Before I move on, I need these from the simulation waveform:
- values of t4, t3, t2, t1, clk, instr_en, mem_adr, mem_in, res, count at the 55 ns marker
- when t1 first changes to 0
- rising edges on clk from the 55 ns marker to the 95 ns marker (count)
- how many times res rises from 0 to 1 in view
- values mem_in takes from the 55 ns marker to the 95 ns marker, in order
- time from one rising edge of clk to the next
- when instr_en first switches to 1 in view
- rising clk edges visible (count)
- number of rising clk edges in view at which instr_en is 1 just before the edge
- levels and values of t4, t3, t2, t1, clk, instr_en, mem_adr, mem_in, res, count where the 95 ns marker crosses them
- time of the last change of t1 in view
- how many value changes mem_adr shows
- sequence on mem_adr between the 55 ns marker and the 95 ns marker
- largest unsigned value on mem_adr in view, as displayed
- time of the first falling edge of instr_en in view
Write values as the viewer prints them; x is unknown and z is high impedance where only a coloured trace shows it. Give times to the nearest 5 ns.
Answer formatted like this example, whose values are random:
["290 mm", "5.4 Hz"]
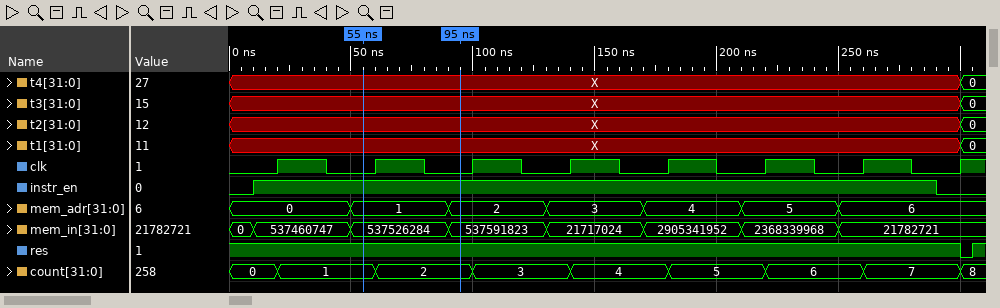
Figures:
["t4=X, t3=X, t2=X, t1=X, clk=0, instr_en=1, mem_adr=1, mem_in=537526284, res=1, count=1", "300 ns", "1", "1", "537526284, 537591823", "40 ns", "10 ns", "8", "7", "t4=X, t3=X, t2=X, t1=X, clk=0, instr_en=1, mem_adr=2, mem_in=537591823, res=1, count=2", "300 ns", "6", "1, 2", "6", "290 ns"]
